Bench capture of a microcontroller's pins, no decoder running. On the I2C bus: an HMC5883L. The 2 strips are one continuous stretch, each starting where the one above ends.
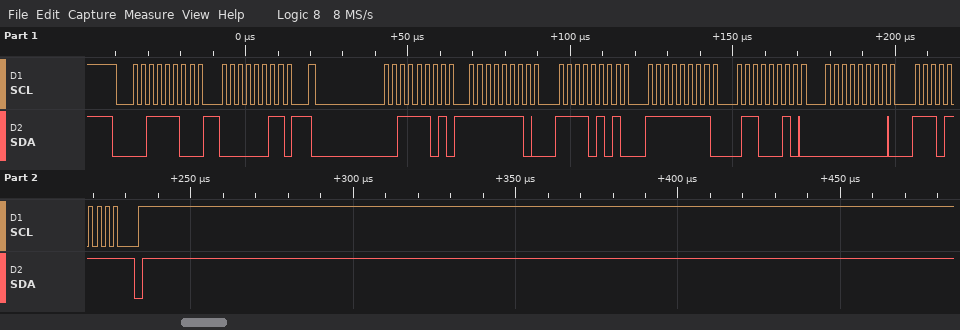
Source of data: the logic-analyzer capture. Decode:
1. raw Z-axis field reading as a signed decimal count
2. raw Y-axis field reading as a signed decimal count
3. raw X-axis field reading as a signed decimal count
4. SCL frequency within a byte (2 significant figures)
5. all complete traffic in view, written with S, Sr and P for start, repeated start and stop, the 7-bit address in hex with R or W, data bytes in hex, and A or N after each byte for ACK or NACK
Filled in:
-158
239
-267
400 kHz
S 1EW A 03 A Sr 1ER A FE A F5 A FF A 62 A 00 A EF N P
